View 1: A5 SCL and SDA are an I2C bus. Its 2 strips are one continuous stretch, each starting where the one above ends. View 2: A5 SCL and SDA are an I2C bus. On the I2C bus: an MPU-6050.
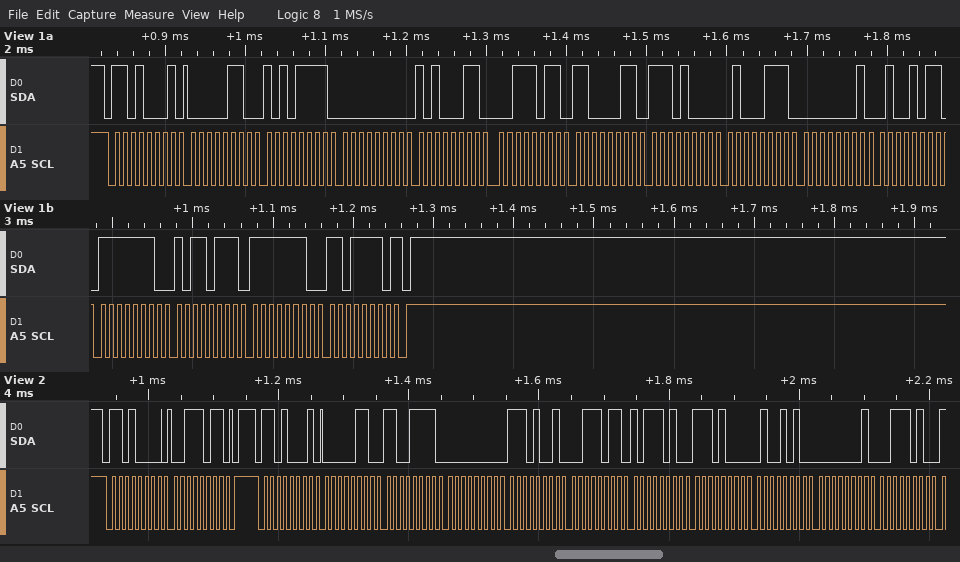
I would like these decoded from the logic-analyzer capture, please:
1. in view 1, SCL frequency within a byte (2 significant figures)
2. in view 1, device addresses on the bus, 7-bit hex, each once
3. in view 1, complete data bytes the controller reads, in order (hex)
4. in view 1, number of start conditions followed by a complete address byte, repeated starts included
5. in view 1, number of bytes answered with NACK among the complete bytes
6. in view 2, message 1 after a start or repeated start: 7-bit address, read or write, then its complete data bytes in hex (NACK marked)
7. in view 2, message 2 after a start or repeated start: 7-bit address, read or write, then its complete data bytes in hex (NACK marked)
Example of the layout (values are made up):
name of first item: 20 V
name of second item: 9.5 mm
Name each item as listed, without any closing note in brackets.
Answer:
in view 1, SCL frequency within a byte: 100 kHz
in view 1, device addresses on the bus, 7-bit hex, each once: 0x68
in view 1, complete data bytes the controller reads, in order: 06 AF 00 A3 3B C3 E8 47 01 4B FE B7 FE DE
in view 1, number of start conditions followed by a complete address byte, repeated starts included: 1
in view 1, number of bytes answered with NACK among the complete bytes: 1
in view 2, message 1 after a start or repeated start: 7-bit address, read or write, then its complete data bytes in hex: 0x68 write: 3B
in view 2, message 2 after a start or repeated start: 7-bit address, read or write, then its complete data bytes in hex: 0x68 read: 06 CF 00 E9 3B BA E8 4A 01 3A
